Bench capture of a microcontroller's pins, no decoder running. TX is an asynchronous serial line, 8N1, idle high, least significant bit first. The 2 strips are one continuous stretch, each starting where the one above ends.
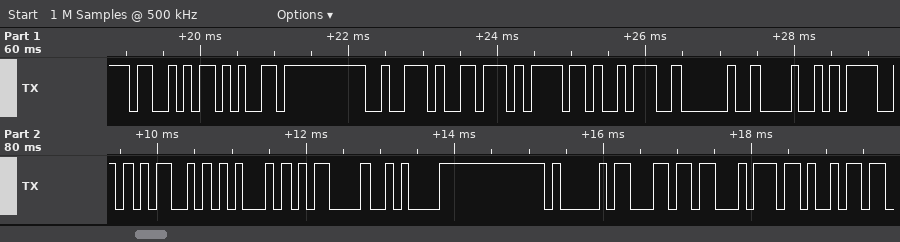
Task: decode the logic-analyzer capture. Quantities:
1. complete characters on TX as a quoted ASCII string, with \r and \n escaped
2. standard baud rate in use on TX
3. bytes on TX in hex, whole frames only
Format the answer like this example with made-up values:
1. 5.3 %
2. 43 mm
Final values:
1. "Servo: HOME\r\nAlti"
2. 9600 baud
3. 53 65 72 76 6F 3A 20 48 4F 4D 45 0D 0A 41 6C 74 69
